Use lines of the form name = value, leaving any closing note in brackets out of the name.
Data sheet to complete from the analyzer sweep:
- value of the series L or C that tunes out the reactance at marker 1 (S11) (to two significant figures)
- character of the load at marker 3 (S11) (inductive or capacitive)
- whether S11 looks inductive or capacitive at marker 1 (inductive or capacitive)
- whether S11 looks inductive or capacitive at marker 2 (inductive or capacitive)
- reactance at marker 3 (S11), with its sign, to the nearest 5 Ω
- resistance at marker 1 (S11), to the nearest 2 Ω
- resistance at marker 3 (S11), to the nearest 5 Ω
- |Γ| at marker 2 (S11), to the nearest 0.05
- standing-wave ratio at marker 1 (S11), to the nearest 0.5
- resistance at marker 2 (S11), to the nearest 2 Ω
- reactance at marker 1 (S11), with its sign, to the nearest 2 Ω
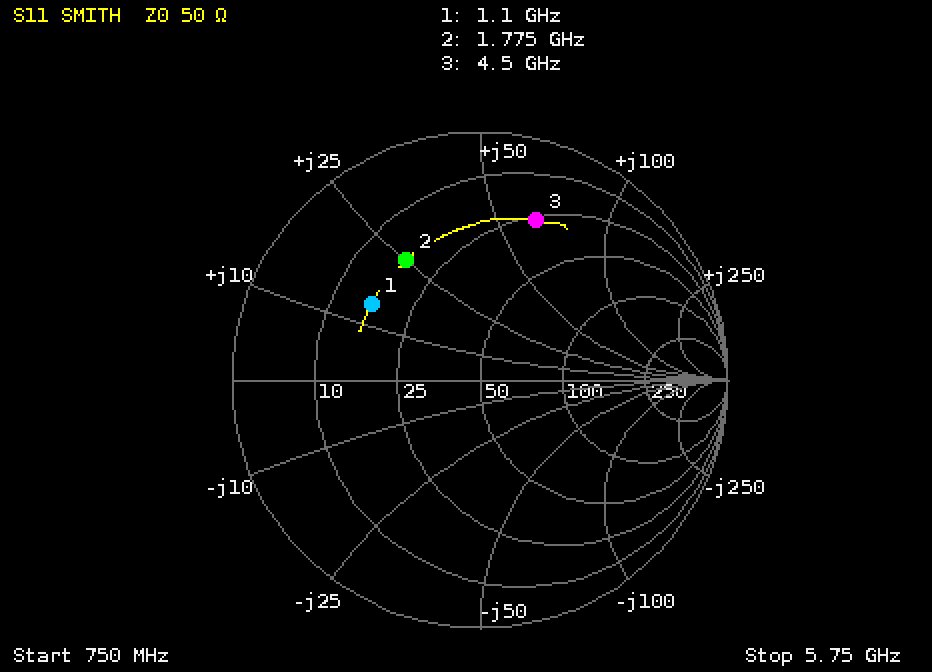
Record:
value of the series L or C that tunes out the reactance at marker 1 (S11) = 10 pF
character of the load at marker 3 (S11) = inductive
whether S11 looks inductive or capacitive at marker 1 = inductive
whether S11 looks inductive or capacitive at marker 2 = inductive
reactance at marker 3 (S11), with its sign, to the nearest 5 Ω = +65 Ω
resistance at marker 1 (S11), to the nearest 2 Ω = 16 Ω
resistance at marker 3 (S11), to the nearest 5 Ω = 25 Ω
|Γ| at marker 2 (S11), to the nearest 0.05 = 0.55
standing-wave ratio at marker 1 (S11), to the nearest 0.5 = 3.5
resistance at marker 2 (S11), to the nearest 2 Ω = 18 Ω
reactance at marker 1 (S11), with its sign, to the nearest 2 Ω = +14 Ω
